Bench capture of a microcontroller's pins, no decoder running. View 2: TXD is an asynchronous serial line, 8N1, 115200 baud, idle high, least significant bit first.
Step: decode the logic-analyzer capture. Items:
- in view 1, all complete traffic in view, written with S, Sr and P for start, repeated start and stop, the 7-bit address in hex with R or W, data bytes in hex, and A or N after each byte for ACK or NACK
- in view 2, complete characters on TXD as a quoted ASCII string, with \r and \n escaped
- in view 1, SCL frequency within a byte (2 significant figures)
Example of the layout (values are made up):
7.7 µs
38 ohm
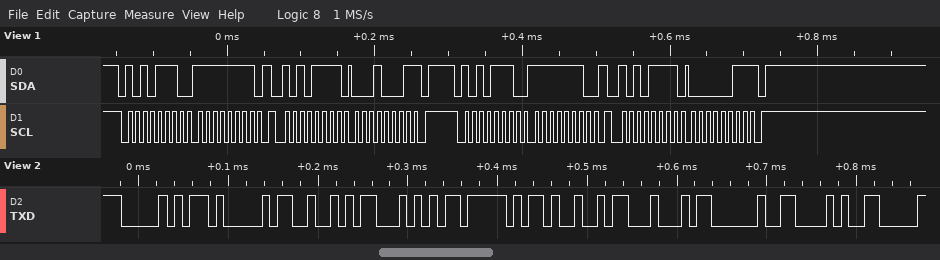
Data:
S 57W A FF A Sr 57R A 11 N P S 57W A FE A Sr 57R A 03 N P
"PART_ID ("
100 kHz
